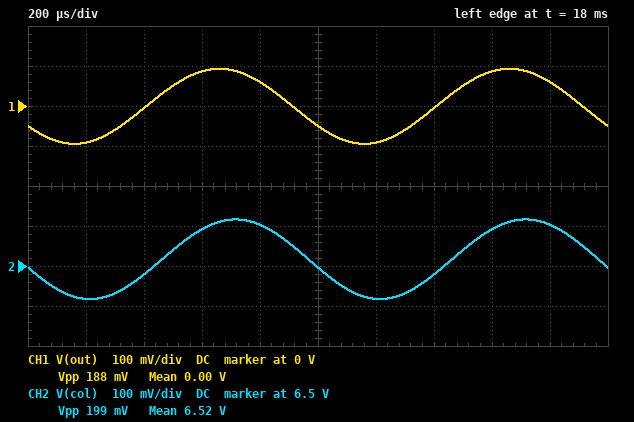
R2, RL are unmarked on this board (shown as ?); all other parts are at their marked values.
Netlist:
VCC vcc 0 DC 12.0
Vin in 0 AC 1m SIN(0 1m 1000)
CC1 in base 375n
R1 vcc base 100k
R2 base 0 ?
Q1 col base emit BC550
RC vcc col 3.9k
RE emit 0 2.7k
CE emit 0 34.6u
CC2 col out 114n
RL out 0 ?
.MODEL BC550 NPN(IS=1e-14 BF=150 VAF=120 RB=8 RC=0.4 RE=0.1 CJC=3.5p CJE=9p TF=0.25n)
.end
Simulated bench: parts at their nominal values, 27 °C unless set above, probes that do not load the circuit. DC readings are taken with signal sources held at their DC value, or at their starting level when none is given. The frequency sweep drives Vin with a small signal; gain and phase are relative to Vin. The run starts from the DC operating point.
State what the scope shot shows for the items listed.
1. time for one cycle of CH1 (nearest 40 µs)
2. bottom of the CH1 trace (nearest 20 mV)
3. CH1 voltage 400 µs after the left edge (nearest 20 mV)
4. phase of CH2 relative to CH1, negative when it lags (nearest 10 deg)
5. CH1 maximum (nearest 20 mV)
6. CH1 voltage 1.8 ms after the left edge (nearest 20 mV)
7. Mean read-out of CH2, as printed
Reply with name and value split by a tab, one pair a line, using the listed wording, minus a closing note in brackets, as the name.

time for one cycle of CH1	1.00 ms
bottom of the CH1 trace	-100 mV
CH1 voltage 400 µs after the left edge	0 V
phase of CH2 relative to CH1, negative when it lags	-20 deg
CH1 maximum	100 mV
CH1 voltage 1.8 ms after the left edge	60 mV
Mean read-out of CH2, as printed	6.52 V
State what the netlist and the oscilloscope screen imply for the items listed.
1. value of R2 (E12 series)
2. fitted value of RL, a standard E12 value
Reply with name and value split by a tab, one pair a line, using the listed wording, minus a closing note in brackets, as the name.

value of R2	68 kΩ
fitted value of RL, a standard E12 value	3.9 kΩ
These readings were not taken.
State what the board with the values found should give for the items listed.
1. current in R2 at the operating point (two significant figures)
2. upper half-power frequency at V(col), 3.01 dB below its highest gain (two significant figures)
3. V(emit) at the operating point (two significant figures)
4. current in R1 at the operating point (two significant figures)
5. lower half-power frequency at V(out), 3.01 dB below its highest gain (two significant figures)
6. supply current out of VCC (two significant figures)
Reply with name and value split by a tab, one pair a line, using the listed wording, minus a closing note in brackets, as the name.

current in R2 at the operating point	66 µA
upper half-power frequency at V(col), 3.01 dB below its highest gain	25 MHz
V(emit) at the operating point	3.8 V
current in R1 at the operating point	75 µA
lower half-power frequency at V(out), 3.01 dB below its highest gain	470 Hz
supply current out of VCC	1.5 mA
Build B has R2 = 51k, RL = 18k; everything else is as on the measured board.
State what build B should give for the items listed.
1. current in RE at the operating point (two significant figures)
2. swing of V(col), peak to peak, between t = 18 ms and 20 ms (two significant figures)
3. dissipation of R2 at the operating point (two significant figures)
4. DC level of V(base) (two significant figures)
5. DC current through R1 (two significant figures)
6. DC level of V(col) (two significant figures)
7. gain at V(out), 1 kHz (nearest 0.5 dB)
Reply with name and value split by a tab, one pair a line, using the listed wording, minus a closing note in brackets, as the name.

current in RE at the operating point	1.2 mA
swing of V(col), peak to peak, between t = 18 ms and 20 ms	260 mV
dissipation of R2 at the operating point	280 µW
DC level of V(base)	3.8 V
DC current through R1	82 µA
DC level of V(col)	7.5 V
gain at V(out), 1 kHz	42.5 dB
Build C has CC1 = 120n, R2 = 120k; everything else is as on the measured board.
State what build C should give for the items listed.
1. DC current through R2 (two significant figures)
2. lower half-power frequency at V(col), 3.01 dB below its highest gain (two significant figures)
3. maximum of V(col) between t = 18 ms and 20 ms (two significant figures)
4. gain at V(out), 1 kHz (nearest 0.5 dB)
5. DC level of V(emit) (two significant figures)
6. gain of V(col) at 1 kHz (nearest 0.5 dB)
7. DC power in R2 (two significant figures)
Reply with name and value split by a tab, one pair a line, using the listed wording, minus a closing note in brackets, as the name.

DC current through R2	46 µA
lower half-power frequency at V(col), 3.01 dB below its highest gain	20 kHz
maximum of V(col) between t = 18 ms and 20 ms	5.0 V
gain at V(out), 1 kHz	9.0 dB
DC level of V(emit)	4.9 V
gain of V(col) at 1 kHz	9.5 dB
DC power in R2	260 µW
